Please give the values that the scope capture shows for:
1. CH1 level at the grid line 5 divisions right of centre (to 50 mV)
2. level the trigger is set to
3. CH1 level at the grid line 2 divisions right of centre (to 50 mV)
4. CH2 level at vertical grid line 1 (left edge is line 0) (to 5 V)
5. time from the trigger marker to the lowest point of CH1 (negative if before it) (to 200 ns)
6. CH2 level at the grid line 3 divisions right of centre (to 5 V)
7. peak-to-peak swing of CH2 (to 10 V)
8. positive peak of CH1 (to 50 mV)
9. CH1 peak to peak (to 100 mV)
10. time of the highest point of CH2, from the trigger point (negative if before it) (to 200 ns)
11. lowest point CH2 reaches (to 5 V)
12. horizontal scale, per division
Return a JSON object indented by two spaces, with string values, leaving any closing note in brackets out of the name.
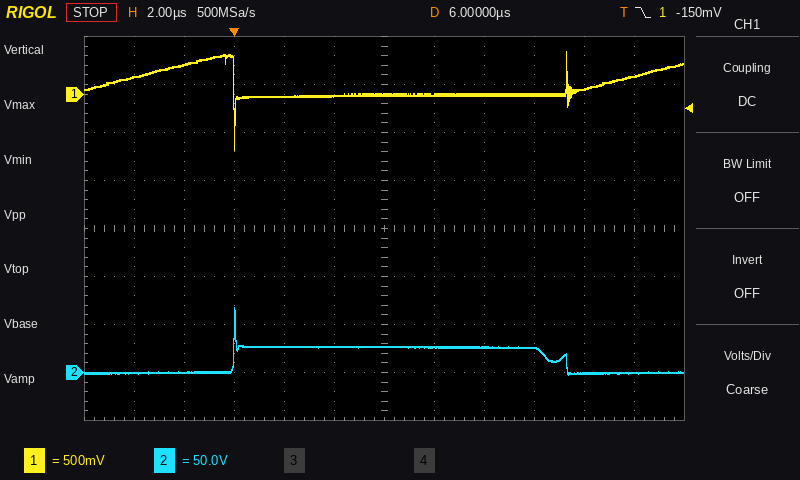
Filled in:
{
  "CH1 level at the grid line 5 divisions right of centre": "200 mV",
  "level the trigger is set to": "-150 mV",
  "CH1 level at the grid line 2 divisions right of centre": "0 mV",
  "CH2 level at vertical grid line 1 (left edge is line 0)": "0 V",
  "time from the trigger marker to the lowest point of CH1 (negative if before it)": "0.0 µs",
  "CH2 level at the grid line 3 divisions right of centre": "25 V",
  "peak-to-peak swing of CH2": "70 V",
  "positive peak of CH1": "450 mV",
  "CH1 peak to peak": "1.00 V",
  "time of the highest point of CH2, from the trigger point (negative if before it)": "0.0 µs",
  "lowest point CH2 reaches": "0 V",
  "horizontal scale, per division": "2 µs"
}
